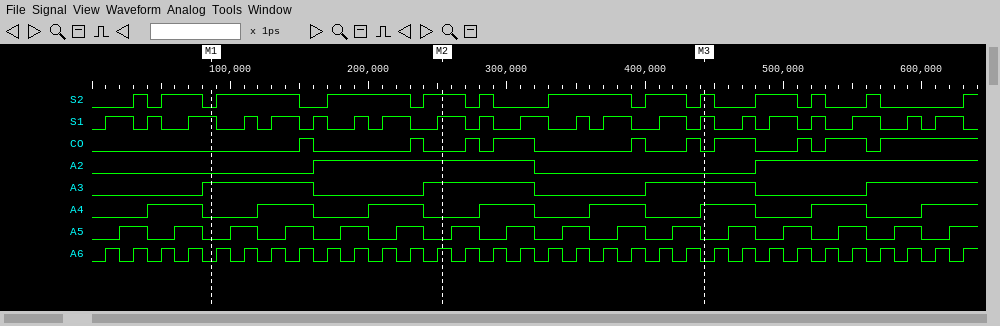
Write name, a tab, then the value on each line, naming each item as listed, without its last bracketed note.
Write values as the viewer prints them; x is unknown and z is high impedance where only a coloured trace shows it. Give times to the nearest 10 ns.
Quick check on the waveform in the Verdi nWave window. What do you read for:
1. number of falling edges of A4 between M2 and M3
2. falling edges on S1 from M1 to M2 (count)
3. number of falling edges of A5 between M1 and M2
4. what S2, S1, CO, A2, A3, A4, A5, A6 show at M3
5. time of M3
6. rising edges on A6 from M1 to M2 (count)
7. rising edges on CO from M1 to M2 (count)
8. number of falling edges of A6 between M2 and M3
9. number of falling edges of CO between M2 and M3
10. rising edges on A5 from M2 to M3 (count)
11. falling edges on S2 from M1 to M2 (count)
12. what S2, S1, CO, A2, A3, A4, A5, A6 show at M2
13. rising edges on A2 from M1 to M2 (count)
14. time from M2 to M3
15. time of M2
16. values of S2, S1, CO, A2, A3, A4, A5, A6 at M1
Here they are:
number of falling edges of A4 between M2 and M3	2
falling edges on S1 from M1 to M2	6
number of falling edges of A5 between M1 and M2	4
what S2, S1, CO, A2, A3, A4, A5, A6 show at M3	S2=1, S1=1, CO=0, A2=0, A3=1, A4=1, A5=0, A6=0
time of M3	440 ns
rising edges on A6 from M1 to M2	9
rising edges on CO from M1 to M2	2
number of falling edges of A6 between M2 and M3	10
number of falling edges of CO between M2 and M3	4
rising edges on A5 from M2 to M3	5
falling edges on S2 from M1 to M2	2
what S2, S1, CO, A2, A3, A4, A5, A6 show at M2	S2=1, S1=1, CO=0, A2=1, A3=1, A4=0, A5=0, A6=1
rising edges on A2 from M1 to M2	1
time from M2 to M3	190 ns
time of M2	250 ns
values of S2, S1, CO, A2, A3, A4, A5, A6 at M1	S2=0, S1=1, CO=0, A2=0, A3=1, A4=0, A5=0, A6=0
